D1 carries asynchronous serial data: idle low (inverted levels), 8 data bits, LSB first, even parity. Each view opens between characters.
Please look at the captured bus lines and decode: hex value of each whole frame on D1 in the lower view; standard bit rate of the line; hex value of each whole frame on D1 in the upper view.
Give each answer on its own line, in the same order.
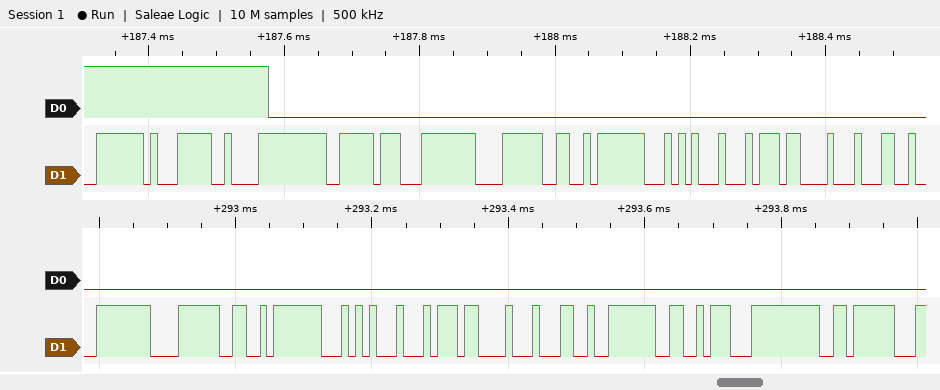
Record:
80, 60, 01, 75, 91, 77, 03, 16, 00, 02
100000 baud
40, B0, 00, 10, 80, 60, 01, 75, 91, 77
